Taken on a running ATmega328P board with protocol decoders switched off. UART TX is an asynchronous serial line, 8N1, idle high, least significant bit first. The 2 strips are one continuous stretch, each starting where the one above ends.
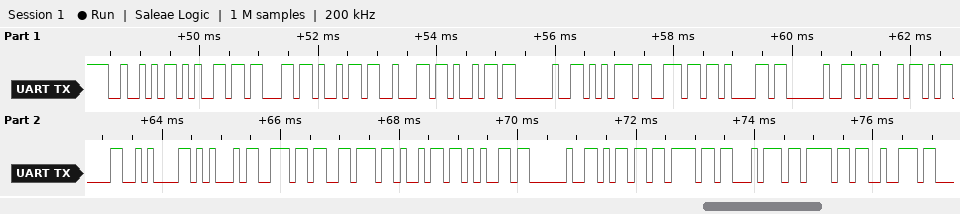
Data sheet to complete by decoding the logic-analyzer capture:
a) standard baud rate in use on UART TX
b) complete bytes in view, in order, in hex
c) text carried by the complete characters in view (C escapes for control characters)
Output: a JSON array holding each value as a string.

["9600 baud", "52 65 63 69 62 69 20 75 6E 61 20 45 0D 0A 45 6E 76 69 65 20 6D 6F 74 6F 72", "\"Recibi una E\\r\\nEnvie motor\""]
